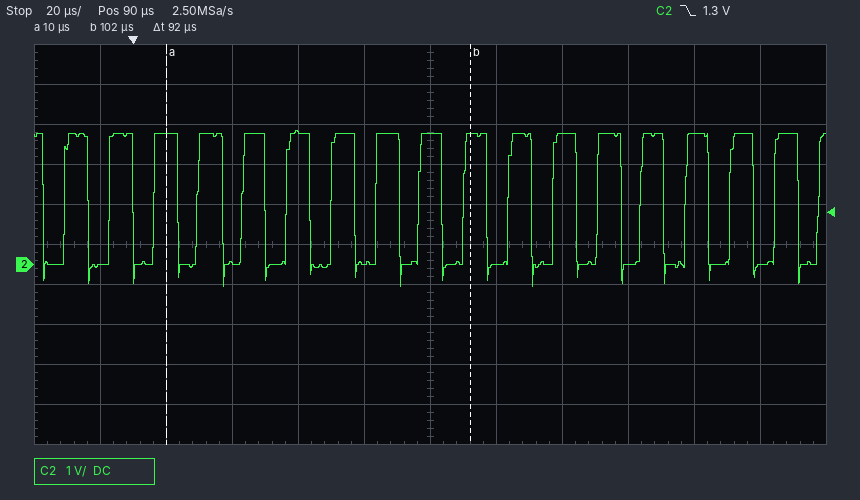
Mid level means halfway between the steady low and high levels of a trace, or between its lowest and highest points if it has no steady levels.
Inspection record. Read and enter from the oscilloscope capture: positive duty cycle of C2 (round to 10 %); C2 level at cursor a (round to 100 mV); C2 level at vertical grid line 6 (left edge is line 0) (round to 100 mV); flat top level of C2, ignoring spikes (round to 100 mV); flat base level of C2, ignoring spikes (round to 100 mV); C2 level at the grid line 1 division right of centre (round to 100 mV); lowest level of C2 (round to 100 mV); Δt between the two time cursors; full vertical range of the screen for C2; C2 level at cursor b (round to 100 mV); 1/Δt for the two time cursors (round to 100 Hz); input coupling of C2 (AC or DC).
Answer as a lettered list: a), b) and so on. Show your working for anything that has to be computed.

a) 50 %
b) 3.3 V
c) 3.3 V
d) 3.3 V
e) 0.0 V
f) 0.0 V
g) -600 mV
h) 92 µs
i) 10 V
j) 3.3 V
k) 1 / 92 µs ≈ 10.9 kHz
l) DC
